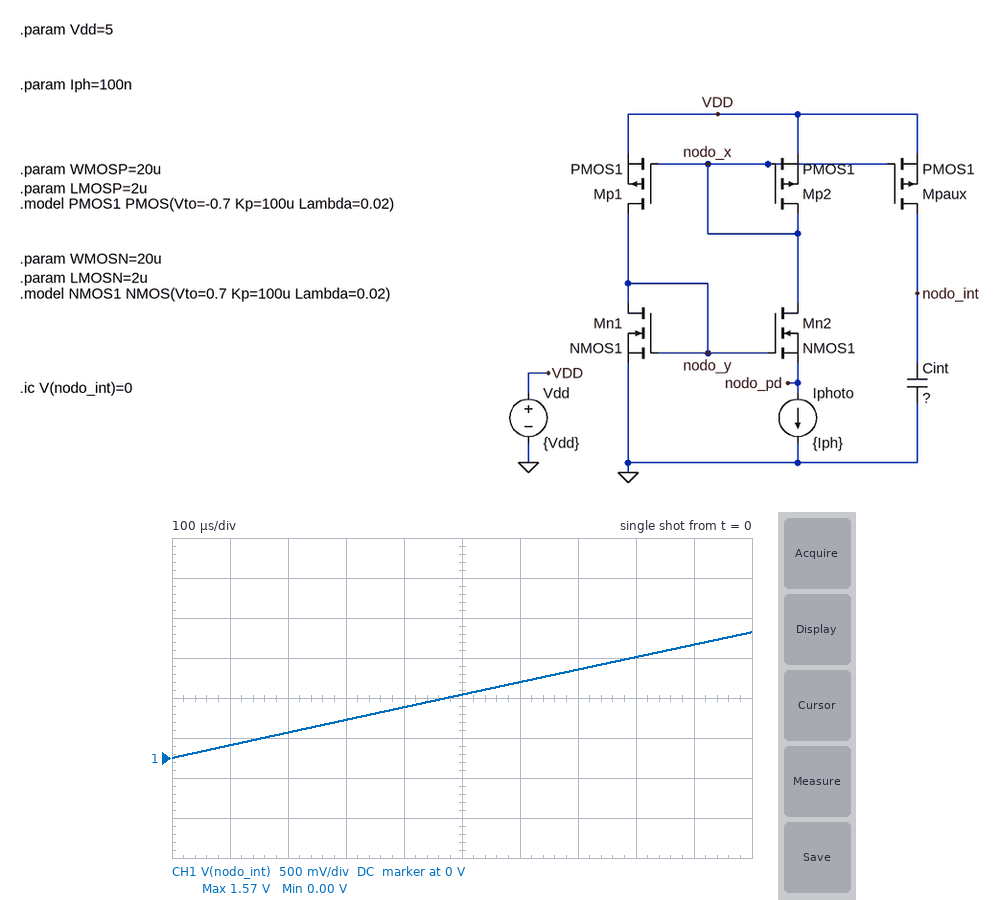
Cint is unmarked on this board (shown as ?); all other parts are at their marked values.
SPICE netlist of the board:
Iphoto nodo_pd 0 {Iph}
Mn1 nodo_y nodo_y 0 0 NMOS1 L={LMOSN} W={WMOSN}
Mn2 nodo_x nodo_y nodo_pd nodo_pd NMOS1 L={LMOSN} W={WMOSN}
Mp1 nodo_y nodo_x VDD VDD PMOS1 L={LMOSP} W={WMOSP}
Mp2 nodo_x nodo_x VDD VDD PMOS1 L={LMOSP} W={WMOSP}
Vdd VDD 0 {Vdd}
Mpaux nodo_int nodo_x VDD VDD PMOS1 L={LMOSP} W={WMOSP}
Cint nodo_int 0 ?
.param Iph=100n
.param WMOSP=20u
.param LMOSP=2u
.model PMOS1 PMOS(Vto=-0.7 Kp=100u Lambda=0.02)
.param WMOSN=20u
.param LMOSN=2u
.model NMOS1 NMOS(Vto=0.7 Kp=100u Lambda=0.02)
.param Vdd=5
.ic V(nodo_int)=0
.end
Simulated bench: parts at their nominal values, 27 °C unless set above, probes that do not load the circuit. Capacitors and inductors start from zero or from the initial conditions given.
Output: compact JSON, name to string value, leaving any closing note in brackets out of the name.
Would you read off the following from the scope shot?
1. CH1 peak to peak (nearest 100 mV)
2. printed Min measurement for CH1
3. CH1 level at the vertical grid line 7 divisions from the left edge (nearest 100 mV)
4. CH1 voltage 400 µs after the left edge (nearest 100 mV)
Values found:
{"CH1 peak to peak": "1.6 V", "printed Min measurement for CH1": "0.00 V", "CH1 level at the vertical grid line 7 divisions from the left edge": "1.1 V", "CH1 voltage 400 µs after the left edge": "600 mV"}
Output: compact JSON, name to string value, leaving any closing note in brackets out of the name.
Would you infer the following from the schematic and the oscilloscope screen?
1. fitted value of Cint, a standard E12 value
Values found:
{"fitted value of Cint, a standard E12 value": "68 pF"}
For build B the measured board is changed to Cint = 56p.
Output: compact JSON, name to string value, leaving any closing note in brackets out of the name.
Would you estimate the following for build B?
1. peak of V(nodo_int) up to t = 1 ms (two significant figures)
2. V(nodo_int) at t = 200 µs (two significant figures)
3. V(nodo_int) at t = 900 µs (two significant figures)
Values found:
{"peak of V(nodo_int) up to t = 1 ms": "1.9 V", "V(nodo_int) at t = 200 µs": "390 mV", "V(nodo_int) at t = 900 µs": "1.7 V"}
